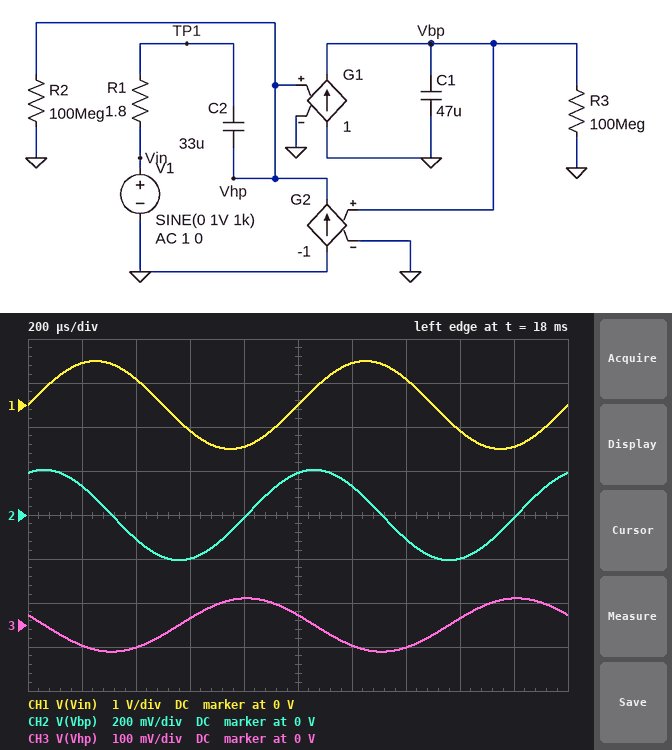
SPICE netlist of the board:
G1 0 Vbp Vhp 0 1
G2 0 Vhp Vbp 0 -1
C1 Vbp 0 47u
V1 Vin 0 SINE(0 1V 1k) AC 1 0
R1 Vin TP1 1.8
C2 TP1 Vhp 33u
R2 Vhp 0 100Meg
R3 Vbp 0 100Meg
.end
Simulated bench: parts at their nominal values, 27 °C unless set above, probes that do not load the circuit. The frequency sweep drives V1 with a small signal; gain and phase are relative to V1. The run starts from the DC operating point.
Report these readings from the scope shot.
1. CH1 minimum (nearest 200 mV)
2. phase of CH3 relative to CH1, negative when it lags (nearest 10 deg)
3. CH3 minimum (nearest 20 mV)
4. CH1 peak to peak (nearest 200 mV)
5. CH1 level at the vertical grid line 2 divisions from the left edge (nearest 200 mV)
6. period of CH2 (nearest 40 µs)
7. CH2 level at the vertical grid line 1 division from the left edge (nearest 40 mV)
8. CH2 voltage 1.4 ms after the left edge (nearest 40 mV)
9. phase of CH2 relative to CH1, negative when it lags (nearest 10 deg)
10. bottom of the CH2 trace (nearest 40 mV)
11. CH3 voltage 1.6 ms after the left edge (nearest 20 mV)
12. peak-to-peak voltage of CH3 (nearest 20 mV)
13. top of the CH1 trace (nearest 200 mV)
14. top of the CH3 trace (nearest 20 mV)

-1.0 V
160 deg
-60 mV
2.0 V
600 mV
1.00 ms
120 mV
-120 mV
70 deg
-200 mV
20 mV
120 mV
1.0 V
60 mV
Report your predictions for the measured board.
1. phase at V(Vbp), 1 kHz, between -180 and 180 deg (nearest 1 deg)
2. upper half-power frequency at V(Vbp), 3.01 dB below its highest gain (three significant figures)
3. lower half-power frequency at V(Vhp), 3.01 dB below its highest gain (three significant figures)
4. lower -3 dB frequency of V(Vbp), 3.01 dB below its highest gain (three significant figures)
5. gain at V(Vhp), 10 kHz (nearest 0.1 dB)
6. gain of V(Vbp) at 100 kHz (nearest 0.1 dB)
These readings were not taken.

68 deg
8.11 kHz
4.33 kHz
2.01 kHz
-0.3 dB
-29.4 dB
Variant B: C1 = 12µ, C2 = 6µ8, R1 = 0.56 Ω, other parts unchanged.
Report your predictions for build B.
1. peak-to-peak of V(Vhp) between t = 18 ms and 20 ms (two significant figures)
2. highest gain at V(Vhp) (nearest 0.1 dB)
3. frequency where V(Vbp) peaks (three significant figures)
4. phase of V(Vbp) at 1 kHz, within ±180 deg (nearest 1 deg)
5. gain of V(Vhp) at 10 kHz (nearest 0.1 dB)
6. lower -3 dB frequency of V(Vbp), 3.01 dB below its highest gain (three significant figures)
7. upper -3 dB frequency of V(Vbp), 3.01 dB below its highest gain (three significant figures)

6.5 mV
7.7 dB
17.6 kHz
89 deg
-7.0 dB
14.3 kHz
21.7 kHz
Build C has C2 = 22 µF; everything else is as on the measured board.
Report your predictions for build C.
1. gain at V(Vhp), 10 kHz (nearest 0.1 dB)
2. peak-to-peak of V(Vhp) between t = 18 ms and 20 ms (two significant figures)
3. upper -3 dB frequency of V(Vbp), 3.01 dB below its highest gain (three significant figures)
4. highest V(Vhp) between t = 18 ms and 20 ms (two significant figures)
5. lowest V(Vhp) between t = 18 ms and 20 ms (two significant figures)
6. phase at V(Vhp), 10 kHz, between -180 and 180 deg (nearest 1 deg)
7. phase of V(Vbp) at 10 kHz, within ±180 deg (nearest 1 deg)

0.3 dB
82 mV
8.86 kHz
41 mV
-41 mV
39 deg
-51 deg
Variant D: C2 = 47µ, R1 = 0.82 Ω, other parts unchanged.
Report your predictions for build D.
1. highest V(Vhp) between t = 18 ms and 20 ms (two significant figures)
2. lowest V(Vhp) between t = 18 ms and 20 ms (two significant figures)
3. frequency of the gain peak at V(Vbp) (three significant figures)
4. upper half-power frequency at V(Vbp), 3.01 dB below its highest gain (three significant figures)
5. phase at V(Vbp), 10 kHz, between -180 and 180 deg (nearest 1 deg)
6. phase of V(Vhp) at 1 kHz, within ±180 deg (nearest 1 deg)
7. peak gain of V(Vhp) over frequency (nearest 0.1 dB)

92 mV
-92 mV
3.39 kHz
5.05 kHz
-73 deg
165 deg
2.5 dB
